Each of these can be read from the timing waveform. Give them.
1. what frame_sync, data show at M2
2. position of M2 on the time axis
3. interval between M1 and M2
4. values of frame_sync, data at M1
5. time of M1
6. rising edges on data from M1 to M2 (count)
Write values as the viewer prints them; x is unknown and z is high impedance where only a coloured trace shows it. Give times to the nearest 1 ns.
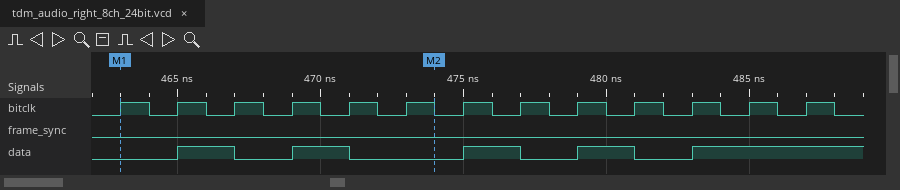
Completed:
frame_sync=0, data=0
474 ns
11 ns
frame_sync=0, data=0
463 ns
2
